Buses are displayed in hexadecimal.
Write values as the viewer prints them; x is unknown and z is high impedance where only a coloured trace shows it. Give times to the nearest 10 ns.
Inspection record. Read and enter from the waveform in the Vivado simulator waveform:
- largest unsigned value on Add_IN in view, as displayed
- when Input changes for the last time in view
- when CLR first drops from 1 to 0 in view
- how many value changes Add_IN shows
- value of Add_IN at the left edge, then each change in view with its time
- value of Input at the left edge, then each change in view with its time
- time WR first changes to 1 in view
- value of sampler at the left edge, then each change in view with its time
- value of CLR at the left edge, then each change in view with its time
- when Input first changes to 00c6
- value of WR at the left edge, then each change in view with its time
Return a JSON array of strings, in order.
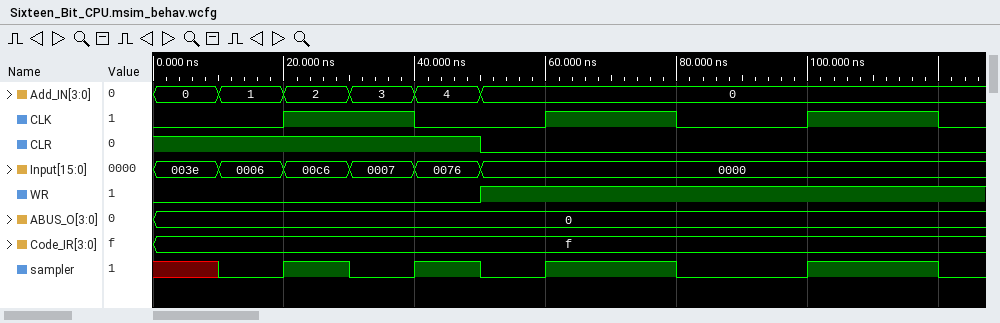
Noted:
["4", "50 ns", "50 ns", "5", "0, 1 at 10 ns, 2 at 20 ns, 3 at 30 ns, 4 at 40 ns, 0 at 50 ns", "003e, 0006 at 10 ns, 00c6 at 20 ns, 0007 at 30 ns, 0076 at 40 ns, 0000 at 50 ns", "50 ns", "x, 0 at 10 ns, 1 at 20 ns, 0 at 30 ns, 1 at 40 ns, 0 at 50 ns, 1 at 60 ns, 0 at 80 ns, 1 at 100 ns, 0 at 120 ns", "1, 0 at 50 ns", "20 ns", "0, 1 at 50 ns"]
